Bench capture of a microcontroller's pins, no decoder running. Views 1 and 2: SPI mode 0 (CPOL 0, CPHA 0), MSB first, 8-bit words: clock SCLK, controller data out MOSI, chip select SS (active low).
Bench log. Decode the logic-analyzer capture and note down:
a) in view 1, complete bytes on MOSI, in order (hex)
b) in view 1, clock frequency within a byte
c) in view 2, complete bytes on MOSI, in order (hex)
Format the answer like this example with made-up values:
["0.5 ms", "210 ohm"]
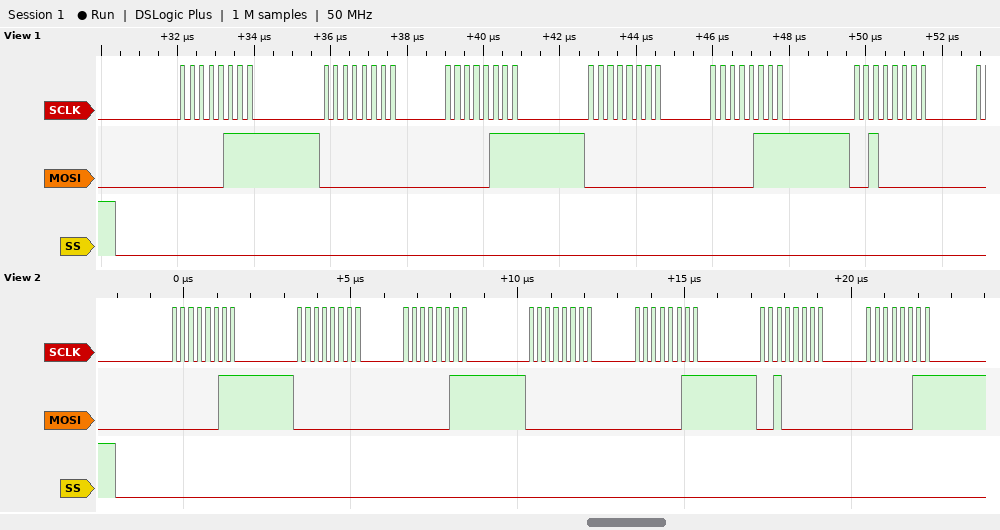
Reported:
["07 00 07 00 07 20", "4 MHz", "03 00 03 00 03 20 03"]
